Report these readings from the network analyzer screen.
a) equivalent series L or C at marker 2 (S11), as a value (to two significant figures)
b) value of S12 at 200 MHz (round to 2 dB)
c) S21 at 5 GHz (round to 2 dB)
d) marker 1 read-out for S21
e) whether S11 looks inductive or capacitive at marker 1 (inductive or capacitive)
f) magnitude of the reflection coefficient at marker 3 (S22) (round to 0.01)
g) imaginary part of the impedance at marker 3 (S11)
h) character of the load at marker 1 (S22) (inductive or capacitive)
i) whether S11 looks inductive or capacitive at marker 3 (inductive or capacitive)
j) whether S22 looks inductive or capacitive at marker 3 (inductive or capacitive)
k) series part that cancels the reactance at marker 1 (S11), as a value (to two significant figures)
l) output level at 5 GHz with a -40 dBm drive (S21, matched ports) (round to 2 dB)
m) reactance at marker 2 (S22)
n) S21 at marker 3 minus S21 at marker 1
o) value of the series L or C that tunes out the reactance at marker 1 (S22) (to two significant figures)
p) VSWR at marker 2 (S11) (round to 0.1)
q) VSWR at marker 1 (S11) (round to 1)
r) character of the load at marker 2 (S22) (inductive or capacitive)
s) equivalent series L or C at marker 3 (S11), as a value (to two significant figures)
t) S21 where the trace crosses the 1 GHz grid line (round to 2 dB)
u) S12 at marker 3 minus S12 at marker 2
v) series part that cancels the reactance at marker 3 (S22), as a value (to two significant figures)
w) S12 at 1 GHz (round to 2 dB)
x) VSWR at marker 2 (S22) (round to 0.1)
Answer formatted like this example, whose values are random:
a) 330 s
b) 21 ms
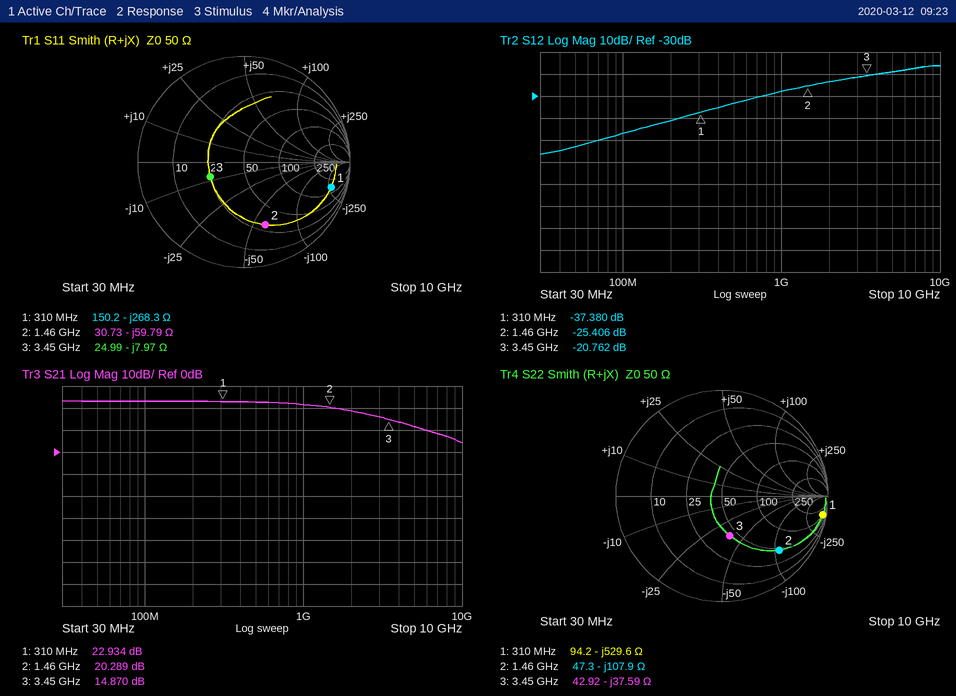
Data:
a) 1.8 pF
b) -42 dB
c) 12 dB
d) 22.934 dB
e) capacitive
f) 0.38
g) -7.97 Ω
h) capacitive
i) capacitive
j) capacitive
k) 140 nH
l) -28 dBm
m) -107.9 Ω
n) -8.064 dB
o) 270 nH
p) 4.3
q) 13
r) capacitive
s) 5.8 pF
t) 22 dB
u) 4.644 dB
v) 1.7 nH
w) -28 dB
x) 6.8
